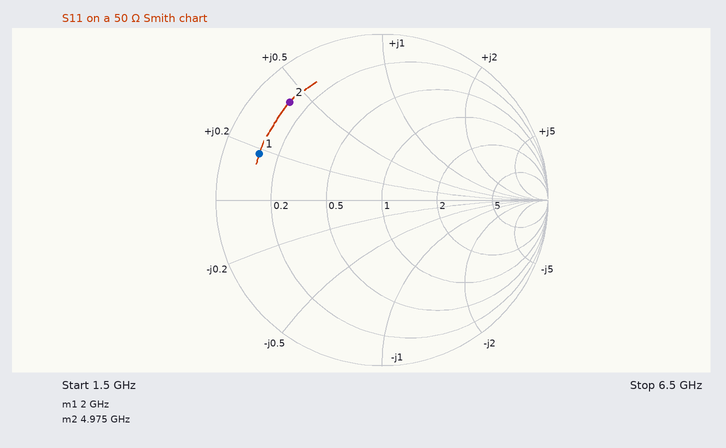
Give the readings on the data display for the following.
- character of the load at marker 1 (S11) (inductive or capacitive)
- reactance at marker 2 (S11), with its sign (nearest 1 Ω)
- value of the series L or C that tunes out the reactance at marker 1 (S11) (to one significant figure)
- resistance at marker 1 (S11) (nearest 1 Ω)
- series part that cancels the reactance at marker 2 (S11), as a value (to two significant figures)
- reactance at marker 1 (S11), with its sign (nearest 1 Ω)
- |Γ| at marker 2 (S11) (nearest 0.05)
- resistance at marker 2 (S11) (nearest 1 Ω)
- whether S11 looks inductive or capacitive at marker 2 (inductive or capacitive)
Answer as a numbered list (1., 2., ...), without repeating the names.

1. inductive
2. +21 Ω
3. 9 pF
4. 6 Ω
5. 1.5 pF
6. +9 Ω
7. 0.80
8. 6 Ω
9. inductive
